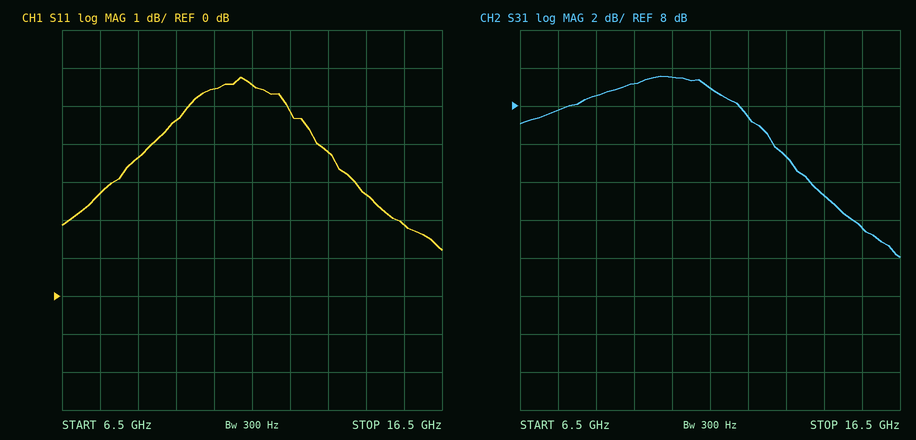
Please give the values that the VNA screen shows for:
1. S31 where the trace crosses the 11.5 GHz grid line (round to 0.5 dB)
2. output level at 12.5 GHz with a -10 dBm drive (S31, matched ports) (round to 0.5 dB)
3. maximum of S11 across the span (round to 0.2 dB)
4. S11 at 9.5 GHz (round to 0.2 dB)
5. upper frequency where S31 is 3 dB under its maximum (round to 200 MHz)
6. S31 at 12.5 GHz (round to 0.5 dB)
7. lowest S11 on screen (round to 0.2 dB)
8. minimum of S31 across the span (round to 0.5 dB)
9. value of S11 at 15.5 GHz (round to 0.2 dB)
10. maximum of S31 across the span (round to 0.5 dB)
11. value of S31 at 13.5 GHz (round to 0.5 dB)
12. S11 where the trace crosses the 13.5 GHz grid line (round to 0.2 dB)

9.0 dB
-2.5 dBm
5.8 dB
4.6 dB
13.0 GHz
7.5 dB
1.2 dB
0.0 dB
1.8 dB
9.5 dB
5.5 dB
3.8 dB
